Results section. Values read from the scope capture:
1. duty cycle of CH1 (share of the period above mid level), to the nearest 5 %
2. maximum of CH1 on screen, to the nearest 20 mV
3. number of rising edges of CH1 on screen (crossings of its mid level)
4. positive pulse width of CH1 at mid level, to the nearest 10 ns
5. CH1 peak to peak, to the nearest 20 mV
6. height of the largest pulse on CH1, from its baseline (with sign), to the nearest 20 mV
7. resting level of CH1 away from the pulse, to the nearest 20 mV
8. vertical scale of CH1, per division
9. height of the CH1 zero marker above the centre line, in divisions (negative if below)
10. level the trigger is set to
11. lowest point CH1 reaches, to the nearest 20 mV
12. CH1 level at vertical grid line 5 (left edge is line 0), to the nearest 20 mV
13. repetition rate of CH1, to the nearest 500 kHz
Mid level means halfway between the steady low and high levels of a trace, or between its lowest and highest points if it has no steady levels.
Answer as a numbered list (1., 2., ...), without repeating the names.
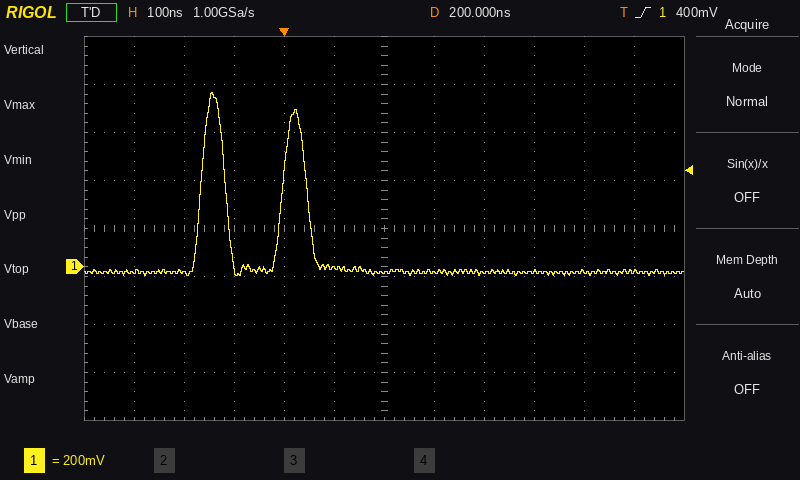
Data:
1. 30 %
2. 720 mV
3. 2
4. 50 ns
5. 760 mV
6. +740 mV
7. -20 mV
8. 200 mV
9. -0.8 div
10. 400 mV
11. -40 mV
12. 0 mV
13. 6.0 MHz
